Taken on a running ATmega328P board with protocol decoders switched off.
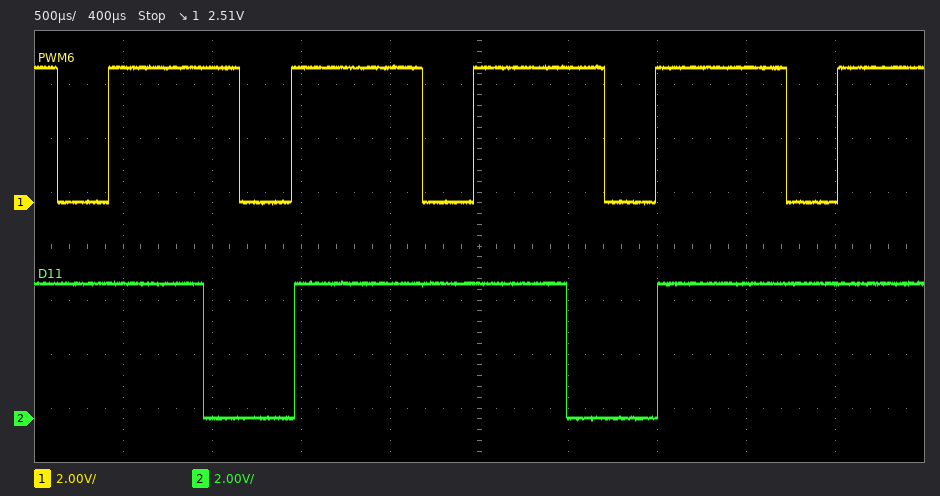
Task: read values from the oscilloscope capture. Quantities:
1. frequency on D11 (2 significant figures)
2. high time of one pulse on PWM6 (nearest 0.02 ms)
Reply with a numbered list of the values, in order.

1. 490 Hz
2. 0.74 ms
